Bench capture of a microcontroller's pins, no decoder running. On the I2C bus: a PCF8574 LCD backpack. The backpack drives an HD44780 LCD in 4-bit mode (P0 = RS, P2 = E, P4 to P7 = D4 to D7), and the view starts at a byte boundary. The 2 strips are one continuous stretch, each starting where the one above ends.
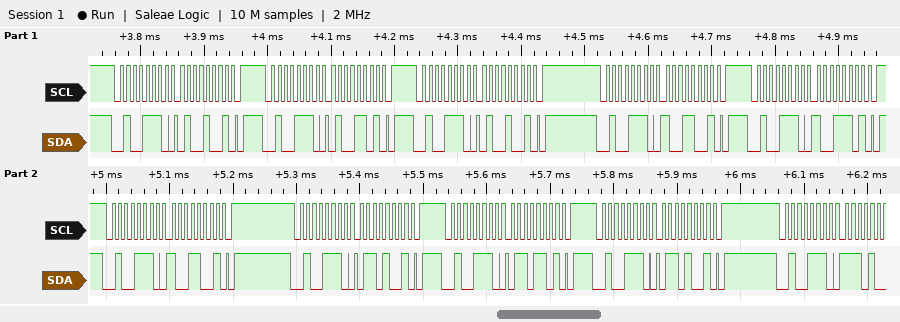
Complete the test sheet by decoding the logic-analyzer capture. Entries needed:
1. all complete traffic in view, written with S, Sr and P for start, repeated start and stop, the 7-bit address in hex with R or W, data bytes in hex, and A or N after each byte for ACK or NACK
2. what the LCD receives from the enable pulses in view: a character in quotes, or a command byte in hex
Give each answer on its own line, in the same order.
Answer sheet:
S 27W A 49 A P S 27W A 4D A P S 27W A 49 A P S 27W A 99 A P S 27W A 9D A P S 27W A 99 A P S 27W A 69 A P S 27W A 6D A P S 27W A 69 A P S 27W A
'I'
